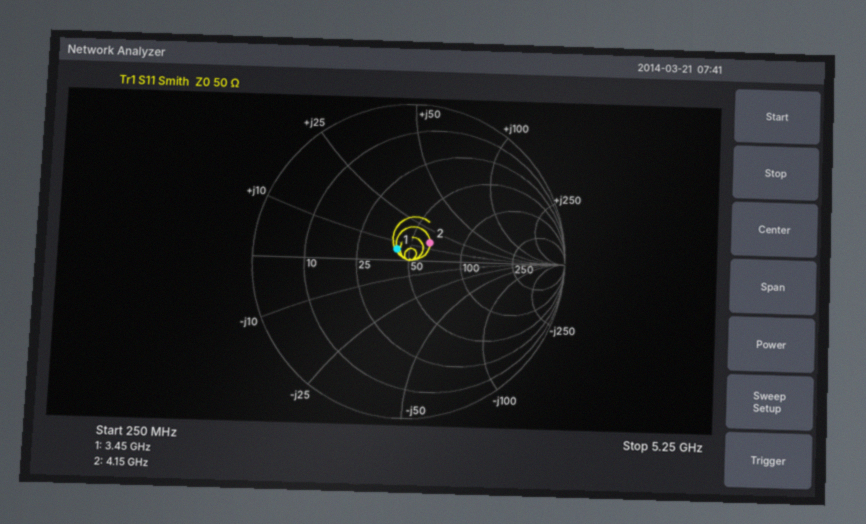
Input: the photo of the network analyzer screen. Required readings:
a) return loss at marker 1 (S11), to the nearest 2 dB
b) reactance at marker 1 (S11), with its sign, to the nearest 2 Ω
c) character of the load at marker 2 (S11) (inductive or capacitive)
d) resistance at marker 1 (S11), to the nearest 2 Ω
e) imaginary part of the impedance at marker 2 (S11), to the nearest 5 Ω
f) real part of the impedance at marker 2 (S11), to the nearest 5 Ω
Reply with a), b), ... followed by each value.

a) 20 dB
b) +6 Ω
c) inductive
d) 42 Ω
e) +15 Ω
f) 65 Ω
